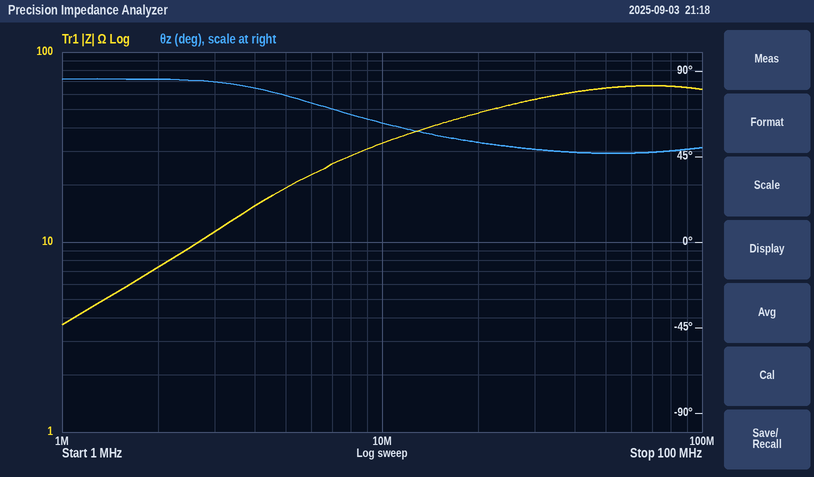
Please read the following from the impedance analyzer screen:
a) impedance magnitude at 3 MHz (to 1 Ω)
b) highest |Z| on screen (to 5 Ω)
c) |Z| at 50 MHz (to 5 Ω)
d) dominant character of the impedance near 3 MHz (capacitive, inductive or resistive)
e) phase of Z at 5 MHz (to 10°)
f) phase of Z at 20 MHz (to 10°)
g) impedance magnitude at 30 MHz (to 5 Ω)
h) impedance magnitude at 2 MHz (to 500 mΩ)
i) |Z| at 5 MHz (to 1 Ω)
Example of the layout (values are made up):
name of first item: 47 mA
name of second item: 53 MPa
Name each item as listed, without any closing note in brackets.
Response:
impedance magnitude at 3 MHz: 11 Ω
highest |Z| on screen: 65 Ω
|Z| at 50 MHz: 65 Ω
dominant character of the impedance near 3 MHz: inductive
phase of Z at 5 MHz: 80°
phase of Z at 20 MHz: 50°
impedance magnitude at 30 MHz: 55 Ω
impedance magnitude at 2 MHz: 7.5 Ω
|Z| at 5 MHz: 19 Ω
